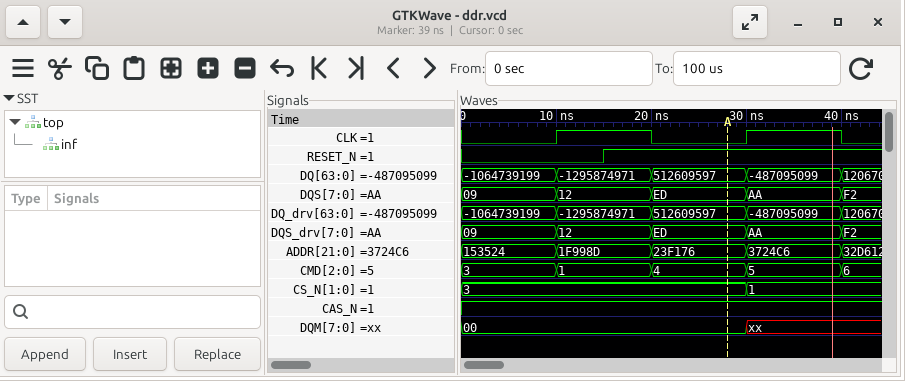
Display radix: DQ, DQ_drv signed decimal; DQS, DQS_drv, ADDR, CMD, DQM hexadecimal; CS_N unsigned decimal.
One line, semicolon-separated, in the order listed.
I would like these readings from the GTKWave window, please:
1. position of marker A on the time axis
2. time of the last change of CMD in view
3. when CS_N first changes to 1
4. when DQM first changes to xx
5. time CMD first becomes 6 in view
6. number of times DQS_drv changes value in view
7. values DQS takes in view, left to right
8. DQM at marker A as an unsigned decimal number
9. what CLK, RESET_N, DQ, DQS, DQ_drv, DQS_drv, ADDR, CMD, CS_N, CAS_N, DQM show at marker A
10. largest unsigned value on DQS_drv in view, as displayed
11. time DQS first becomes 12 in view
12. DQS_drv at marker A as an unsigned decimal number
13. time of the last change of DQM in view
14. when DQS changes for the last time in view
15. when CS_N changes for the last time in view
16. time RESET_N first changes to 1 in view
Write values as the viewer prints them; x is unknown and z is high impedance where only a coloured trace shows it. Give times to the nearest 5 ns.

30 ns; 40 ns; 30 ns; 30 ns; 40 ns; 4; 09, 12, ED, AA, F2; 0; CLK=0, RESET_N=1, DQ=512609597, DQS=ED, DQ_drv=512609597, DQS_drv=ED, ADDR=23F176, CMD=4, CS_N=3, CAS_N=1, DQM=00; F2; 10 ns; 237; 30 ns; 40 ns; 30 ns; 15 ns
